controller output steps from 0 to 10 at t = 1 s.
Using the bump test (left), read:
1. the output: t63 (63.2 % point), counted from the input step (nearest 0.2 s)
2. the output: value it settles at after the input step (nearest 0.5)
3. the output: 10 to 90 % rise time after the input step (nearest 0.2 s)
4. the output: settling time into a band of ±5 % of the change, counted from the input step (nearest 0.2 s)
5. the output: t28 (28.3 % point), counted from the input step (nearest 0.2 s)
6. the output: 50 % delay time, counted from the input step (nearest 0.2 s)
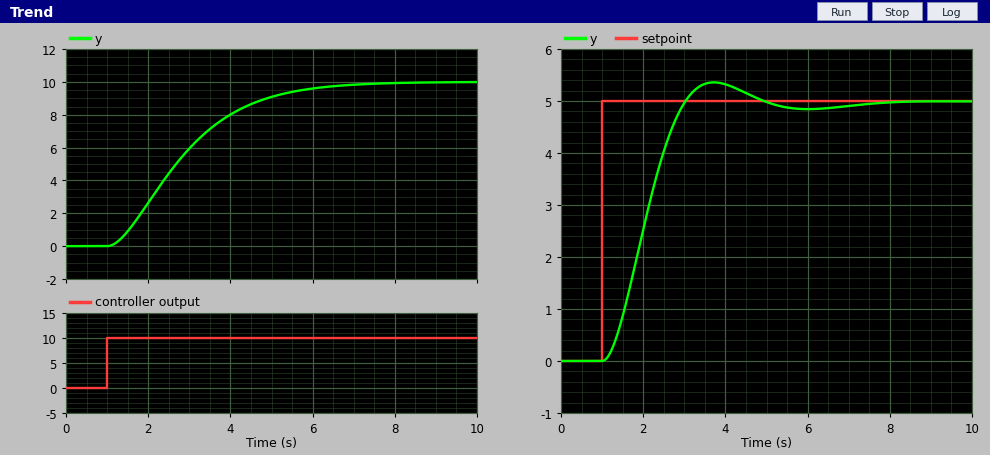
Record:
2.2 s
10.0
3.4 s
4.8 s
1.0 s
1.6 s
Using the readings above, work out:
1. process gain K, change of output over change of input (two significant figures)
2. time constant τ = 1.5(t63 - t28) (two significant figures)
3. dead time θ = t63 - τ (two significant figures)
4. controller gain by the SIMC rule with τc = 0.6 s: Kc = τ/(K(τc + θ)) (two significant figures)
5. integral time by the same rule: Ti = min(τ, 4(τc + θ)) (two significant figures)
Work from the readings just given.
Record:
1.0
1.8 s
0.40 s
1.8
1.8 s
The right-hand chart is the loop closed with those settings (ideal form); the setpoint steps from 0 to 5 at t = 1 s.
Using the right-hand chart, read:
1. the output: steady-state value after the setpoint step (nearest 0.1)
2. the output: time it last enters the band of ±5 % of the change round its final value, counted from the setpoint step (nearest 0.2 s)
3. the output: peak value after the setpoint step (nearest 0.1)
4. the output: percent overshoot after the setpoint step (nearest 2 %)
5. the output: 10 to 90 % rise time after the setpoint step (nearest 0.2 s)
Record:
5.0
3.2 s
5.4
8 %
1.4 s
